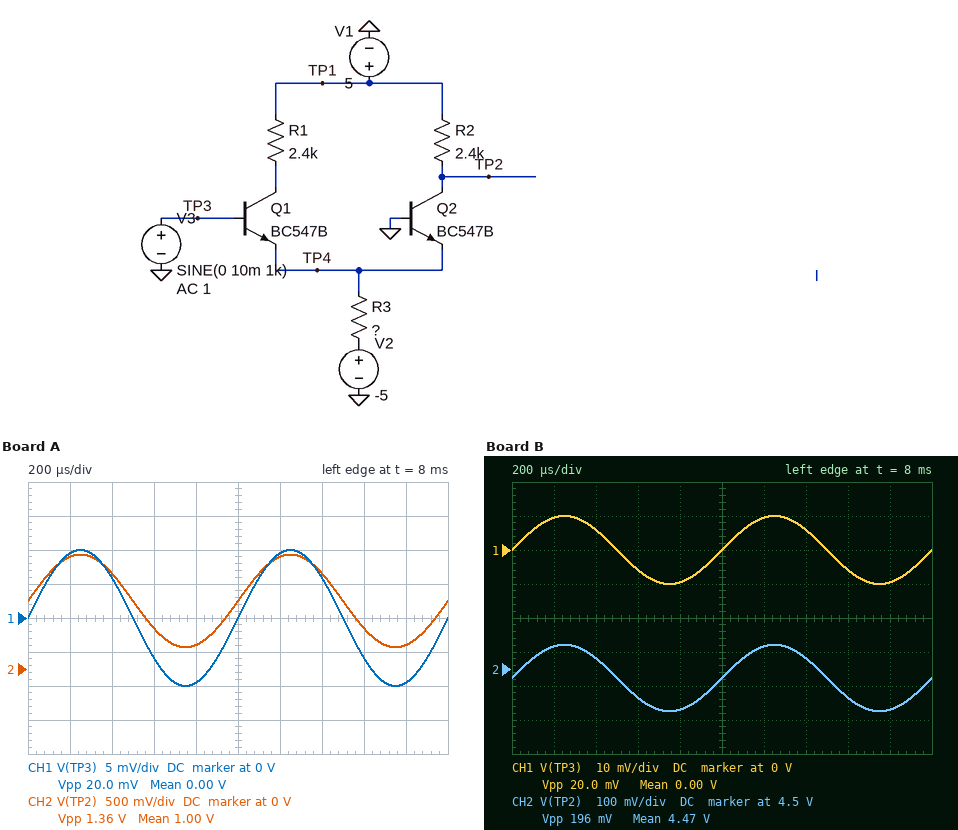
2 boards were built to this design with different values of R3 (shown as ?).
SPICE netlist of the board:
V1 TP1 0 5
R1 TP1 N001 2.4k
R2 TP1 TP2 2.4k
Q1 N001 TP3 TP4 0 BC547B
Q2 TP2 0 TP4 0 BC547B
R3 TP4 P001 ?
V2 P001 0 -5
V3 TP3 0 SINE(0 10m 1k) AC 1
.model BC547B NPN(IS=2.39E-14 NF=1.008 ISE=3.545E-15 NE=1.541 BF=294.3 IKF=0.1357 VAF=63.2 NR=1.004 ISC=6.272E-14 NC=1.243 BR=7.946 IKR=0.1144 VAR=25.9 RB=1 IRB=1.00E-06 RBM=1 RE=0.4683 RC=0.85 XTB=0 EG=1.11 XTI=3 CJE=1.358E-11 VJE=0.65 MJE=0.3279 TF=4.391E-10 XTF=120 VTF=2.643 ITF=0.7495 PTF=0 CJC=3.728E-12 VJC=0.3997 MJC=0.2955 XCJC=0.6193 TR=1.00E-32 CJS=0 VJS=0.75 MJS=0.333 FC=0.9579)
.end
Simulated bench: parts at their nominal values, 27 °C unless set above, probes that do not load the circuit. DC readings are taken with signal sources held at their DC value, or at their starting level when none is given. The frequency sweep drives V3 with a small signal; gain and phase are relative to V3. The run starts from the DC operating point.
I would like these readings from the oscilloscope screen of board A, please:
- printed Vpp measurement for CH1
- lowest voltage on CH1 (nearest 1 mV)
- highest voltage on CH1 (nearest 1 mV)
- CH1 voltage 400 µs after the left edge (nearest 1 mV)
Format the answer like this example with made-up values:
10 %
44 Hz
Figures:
20.0 mV
-10 mV
10 mV
6 mV
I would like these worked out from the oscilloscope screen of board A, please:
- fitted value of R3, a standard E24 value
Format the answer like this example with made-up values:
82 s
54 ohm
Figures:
1.3 kΩ
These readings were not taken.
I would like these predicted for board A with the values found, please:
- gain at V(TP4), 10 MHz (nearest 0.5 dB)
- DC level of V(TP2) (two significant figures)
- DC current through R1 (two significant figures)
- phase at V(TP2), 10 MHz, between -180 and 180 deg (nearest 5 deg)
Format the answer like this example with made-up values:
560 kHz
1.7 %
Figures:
-6.0 dB
1.0 V
1.7 mA
-20 deg
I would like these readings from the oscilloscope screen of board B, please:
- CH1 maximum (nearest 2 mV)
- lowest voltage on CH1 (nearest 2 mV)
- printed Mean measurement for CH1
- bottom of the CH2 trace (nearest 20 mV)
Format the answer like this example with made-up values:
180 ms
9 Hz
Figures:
10 mV
-10 mV
0.00 V
4.38 V
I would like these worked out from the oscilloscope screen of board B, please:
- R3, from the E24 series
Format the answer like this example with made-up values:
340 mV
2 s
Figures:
10 kΩ
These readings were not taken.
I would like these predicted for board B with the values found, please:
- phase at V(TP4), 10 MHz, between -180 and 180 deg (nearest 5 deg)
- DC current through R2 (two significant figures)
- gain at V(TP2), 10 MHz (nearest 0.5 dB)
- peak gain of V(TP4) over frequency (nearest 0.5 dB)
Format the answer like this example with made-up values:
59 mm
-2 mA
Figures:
0 deg
220 µA
19.5 dB
-6.0 dB
